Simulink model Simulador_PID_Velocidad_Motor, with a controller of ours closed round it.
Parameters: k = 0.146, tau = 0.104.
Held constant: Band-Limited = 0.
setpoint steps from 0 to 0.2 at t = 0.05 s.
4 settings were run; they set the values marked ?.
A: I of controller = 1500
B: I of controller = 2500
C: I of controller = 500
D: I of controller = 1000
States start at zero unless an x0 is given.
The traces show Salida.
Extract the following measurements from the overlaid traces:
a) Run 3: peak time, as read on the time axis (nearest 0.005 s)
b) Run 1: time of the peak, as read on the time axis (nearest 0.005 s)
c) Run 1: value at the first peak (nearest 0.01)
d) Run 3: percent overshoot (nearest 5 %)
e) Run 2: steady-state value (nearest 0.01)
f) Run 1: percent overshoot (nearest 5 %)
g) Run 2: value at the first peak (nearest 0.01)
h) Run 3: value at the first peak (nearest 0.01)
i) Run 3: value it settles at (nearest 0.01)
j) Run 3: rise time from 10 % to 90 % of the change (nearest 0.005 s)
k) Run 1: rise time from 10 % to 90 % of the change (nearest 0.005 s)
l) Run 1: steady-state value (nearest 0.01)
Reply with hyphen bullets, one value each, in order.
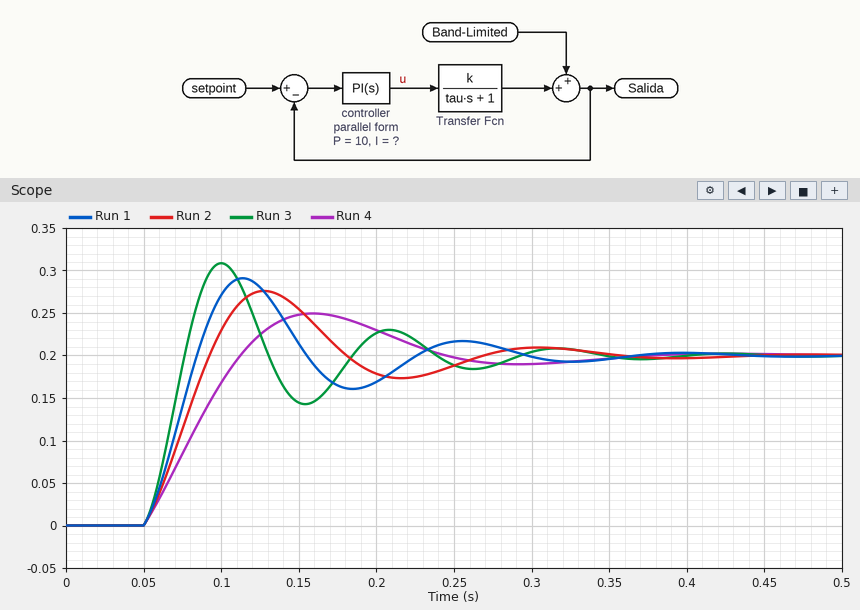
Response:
- 0.100 s
- 0.115 s
- 0.29
- 55 %
- 0.20
- 45 %
- 0.28
- 0.31
- 0.20
- 0.020 s
- 0.025 s
- 0.20
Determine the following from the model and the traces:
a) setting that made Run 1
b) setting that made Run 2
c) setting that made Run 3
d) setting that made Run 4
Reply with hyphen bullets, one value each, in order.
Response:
- A
- D
- B
- C
